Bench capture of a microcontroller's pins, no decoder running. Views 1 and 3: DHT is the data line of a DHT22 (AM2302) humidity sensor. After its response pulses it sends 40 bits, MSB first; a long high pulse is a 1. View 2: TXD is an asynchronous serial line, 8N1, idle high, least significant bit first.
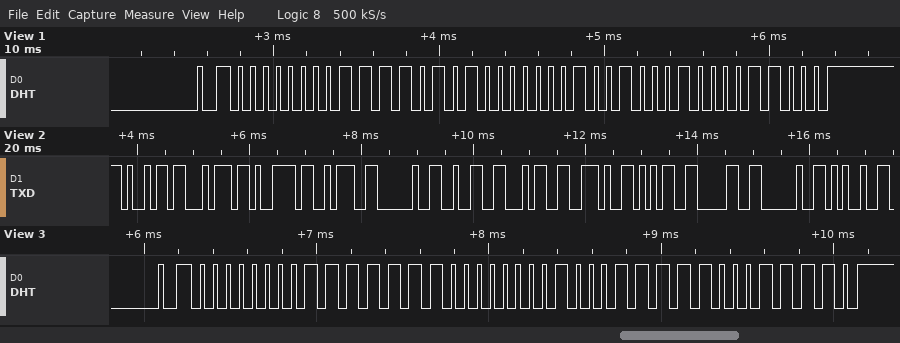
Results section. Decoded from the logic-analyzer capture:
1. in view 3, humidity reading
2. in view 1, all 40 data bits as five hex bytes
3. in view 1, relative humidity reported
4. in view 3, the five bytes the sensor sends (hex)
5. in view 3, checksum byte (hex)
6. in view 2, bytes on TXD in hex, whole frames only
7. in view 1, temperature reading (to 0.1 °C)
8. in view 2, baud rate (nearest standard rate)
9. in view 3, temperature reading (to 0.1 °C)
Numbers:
25.4 %
00 F5 01 22 18
24.5 %
00 FE 01 1F 1E
0x1E
69 74 79 3A 20 32 34 2E 35 30 20 25
29.0 °C
9600 baud
28.7 °C
